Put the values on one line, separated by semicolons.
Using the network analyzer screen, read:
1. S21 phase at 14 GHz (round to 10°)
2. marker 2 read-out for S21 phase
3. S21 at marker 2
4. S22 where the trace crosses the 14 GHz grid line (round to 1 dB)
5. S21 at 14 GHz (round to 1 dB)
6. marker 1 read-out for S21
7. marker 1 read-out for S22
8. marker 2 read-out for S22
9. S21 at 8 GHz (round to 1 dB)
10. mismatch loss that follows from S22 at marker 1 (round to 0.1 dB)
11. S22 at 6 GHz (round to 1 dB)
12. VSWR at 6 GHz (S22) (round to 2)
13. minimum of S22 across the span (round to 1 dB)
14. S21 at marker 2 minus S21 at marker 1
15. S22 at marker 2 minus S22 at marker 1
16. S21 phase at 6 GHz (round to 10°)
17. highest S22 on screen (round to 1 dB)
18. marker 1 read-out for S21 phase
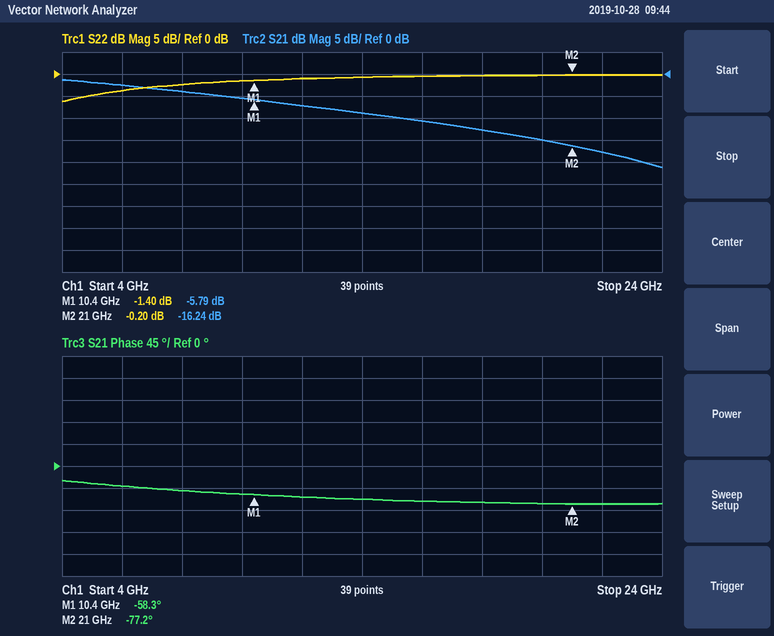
-70°; -77.2°; -16.24 dB; -1 dB; -9 dB; -5.79 dB; -1.40 dB; -0.20 dB; -4 dB; 5.6 dB; -4 dB; 4; -6 dB; -10.45 dB; 1.20 dB; -40°; 0 dB; -58.3°
